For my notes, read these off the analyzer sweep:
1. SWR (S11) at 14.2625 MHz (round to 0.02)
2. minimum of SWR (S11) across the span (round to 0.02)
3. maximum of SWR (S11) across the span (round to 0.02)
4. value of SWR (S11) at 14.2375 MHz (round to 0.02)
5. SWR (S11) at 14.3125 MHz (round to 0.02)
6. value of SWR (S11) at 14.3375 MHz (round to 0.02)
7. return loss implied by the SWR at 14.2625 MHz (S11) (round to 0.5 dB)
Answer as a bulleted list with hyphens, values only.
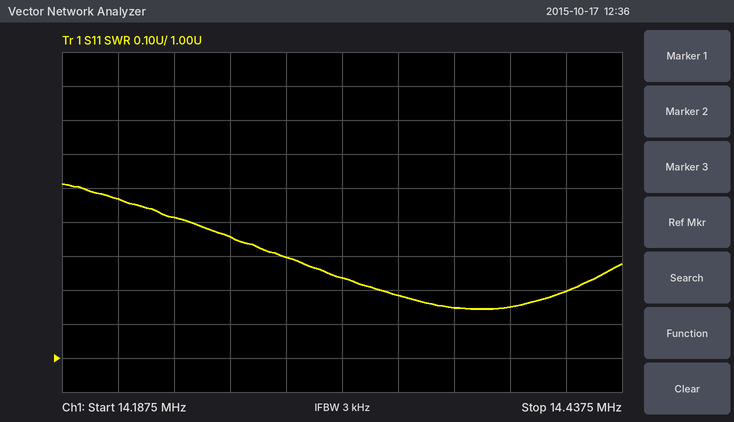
- 1.36
- 1.14
- 1.52
- 1.42
- 1.24
- 1.18
- 16.5 dB
